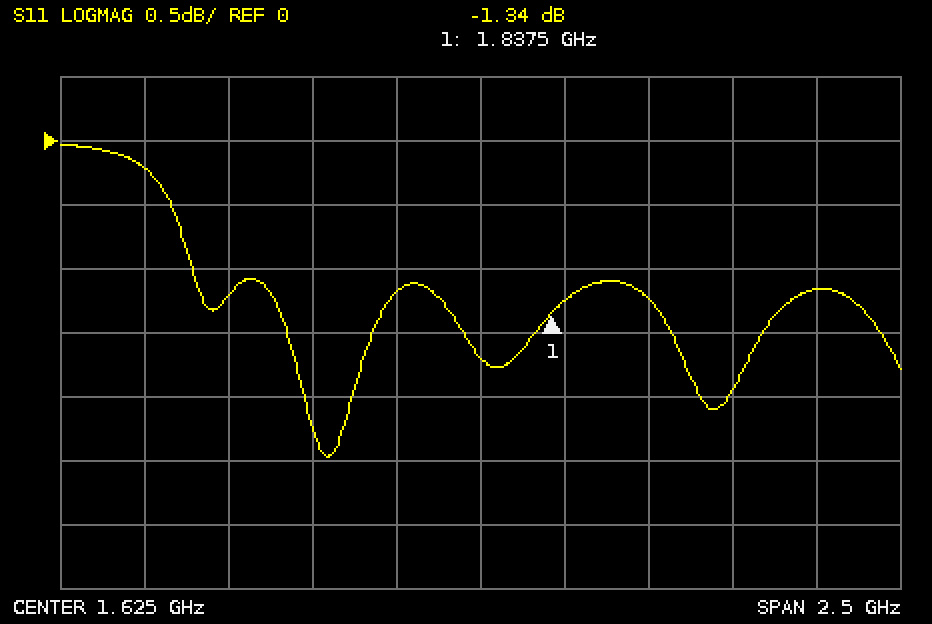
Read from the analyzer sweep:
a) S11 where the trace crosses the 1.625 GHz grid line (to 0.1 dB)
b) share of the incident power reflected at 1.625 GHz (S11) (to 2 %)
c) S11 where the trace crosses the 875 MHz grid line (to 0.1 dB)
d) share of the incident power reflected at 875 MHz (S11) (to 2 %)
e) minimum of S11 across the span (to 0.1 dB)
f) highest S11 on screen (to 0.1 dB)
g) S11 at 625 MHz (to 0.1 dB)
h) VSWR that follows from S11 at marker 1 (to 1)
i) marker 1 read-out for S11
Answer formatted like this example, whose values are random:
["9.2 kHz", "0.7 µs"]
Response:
["-1.7 dB", "68 %", "-1.2 dB", "76 %", "-2.5 dB", "0.0 dB", "-0.2 dB", "13", "-1.34 dB"]
